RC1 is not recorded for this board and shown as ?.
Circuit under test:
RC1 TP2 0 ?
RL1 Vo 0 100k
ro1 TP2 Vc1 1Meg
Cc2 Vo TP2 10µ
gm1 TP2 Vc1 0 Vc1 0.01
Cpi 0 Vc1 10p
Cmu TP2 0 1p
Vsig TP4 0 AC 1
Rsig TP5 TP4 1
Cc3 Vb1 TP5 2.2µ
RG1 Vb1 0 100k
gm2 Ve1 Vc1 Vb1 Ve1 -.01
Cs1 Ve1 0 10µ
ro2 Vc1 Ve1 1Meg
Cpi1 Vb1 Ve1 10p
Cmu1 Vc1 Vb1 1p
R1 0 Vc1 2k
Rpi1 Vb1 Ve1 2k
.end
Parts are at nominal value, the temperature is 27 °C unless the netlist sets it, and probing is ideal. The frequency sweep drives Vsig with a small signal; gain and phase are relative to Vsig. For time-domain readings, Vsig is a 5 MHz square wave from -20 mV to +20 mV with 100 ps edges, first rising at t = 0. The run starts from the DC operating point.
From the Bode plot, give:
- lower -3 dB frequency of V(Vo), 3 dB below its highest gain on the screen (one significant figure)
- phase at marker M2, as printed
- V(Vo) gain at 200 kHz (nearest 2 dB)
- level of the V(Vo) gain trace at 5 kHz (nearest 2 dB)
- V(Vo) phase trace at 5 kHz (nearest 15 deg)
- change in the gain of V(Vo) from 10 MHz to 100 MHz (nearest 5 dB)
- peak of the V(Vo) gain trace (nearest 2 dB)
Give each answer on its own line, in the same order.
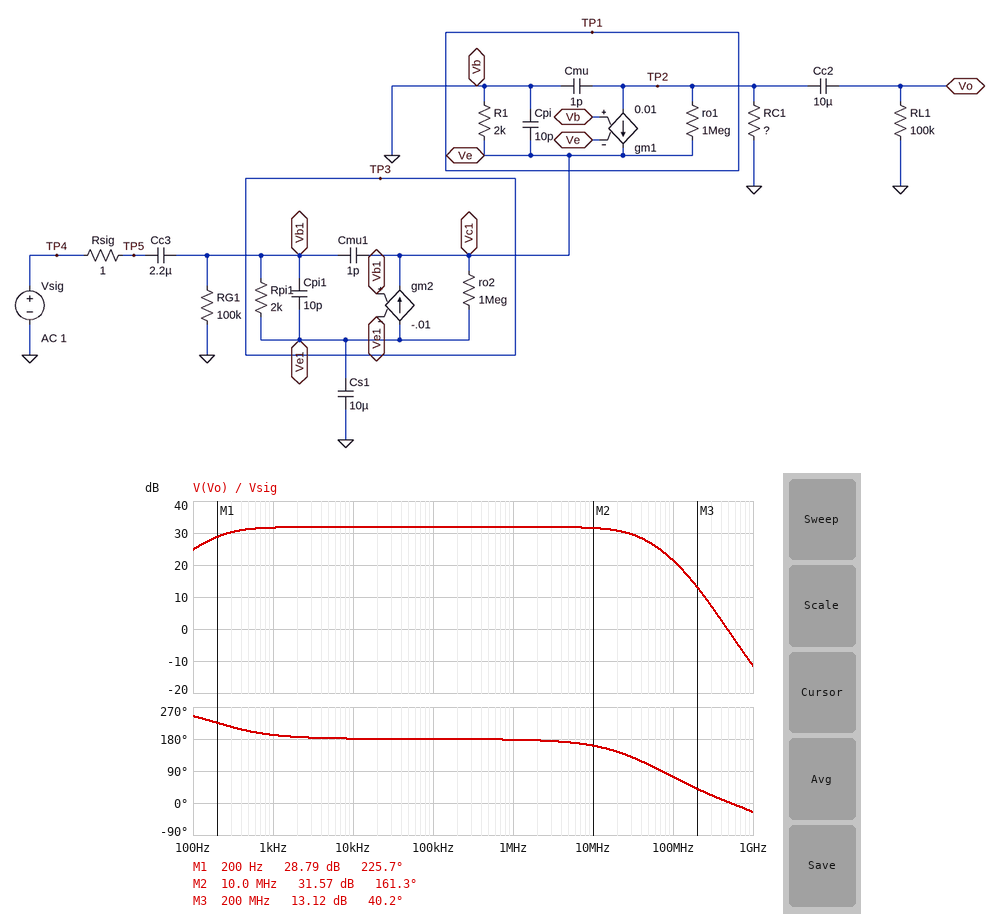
200 Hz
161.3 deg
32 dB
32 dB
180 deg
-10 dB
32 dB
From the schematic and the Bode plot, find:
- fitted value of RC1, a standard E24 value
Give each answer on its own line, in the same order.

4.3 kΩ
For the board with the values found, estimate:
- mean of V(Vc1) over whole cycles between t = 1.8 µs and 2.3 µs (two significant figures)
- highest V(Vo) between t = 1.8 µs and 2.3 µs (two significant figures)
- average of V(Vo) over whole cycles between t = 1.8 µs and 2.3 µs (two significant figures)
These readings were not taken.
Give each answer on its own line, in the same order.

-19 mV
3.7 mV
-780 mV
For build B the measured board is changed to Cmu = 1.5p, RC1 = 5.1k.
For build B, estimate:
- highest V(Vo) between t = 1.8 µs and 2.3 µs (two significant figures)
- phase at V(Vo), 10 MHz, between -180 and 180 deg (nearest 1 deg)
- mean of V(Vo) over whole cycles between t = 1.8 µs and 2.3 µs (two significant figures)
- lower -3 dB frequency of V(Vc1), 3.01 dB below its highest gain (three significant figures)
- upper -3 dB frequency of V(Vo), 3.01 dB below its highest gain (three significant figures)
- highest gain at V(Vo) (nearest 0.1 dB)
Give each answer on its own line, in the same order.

3.6 mV
151 deg
-920 mV
203 Hz
21.4 MHz
33.3 dB
